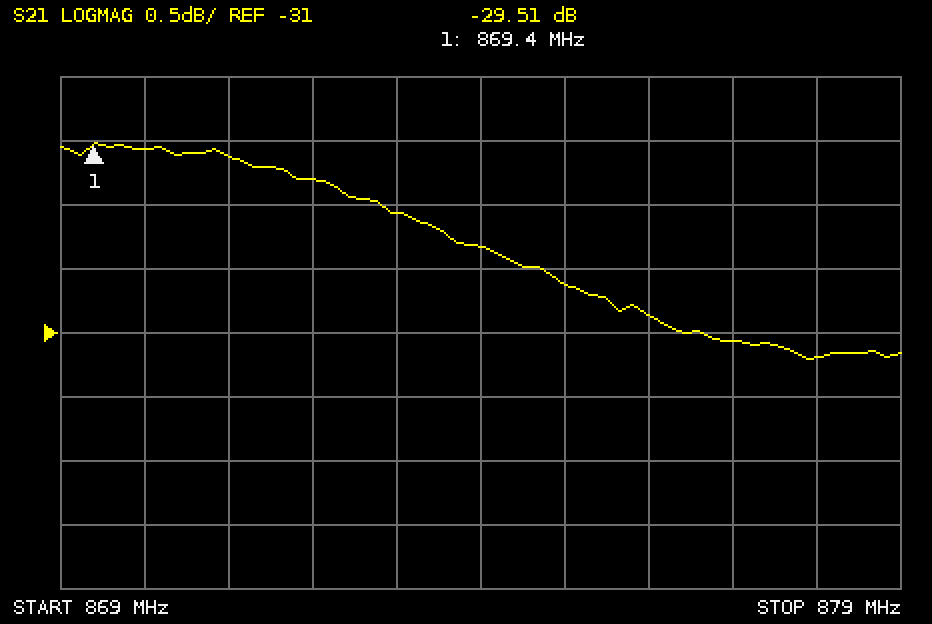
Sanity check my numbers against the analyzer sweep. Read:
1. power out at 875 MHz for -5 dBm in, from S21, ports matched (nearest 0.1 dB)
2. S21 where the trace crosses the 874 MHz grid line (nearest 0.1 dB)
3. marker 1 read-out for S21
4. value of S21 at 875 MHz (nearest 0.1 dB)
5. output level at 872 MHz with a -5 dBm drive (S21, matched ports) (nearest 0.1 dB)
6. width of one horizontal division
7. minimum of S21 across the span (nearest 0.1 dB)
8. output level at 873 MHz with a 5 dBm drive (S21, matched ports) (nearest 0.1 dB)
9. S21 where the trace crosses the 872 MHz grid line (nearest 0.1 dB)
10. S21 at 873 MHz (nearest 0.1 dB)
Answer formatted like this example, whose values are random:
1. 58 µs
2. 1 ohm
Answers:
1. -35.6 dBm
2. -30.3 dB
3. -29.51 dB
4. -30.6 dB
5. -34.8 dBm
6. 1 MHz
7. -31.2 dB
8. -25.1 dBm
9. -29.8 dB
10. -30.1 dB
